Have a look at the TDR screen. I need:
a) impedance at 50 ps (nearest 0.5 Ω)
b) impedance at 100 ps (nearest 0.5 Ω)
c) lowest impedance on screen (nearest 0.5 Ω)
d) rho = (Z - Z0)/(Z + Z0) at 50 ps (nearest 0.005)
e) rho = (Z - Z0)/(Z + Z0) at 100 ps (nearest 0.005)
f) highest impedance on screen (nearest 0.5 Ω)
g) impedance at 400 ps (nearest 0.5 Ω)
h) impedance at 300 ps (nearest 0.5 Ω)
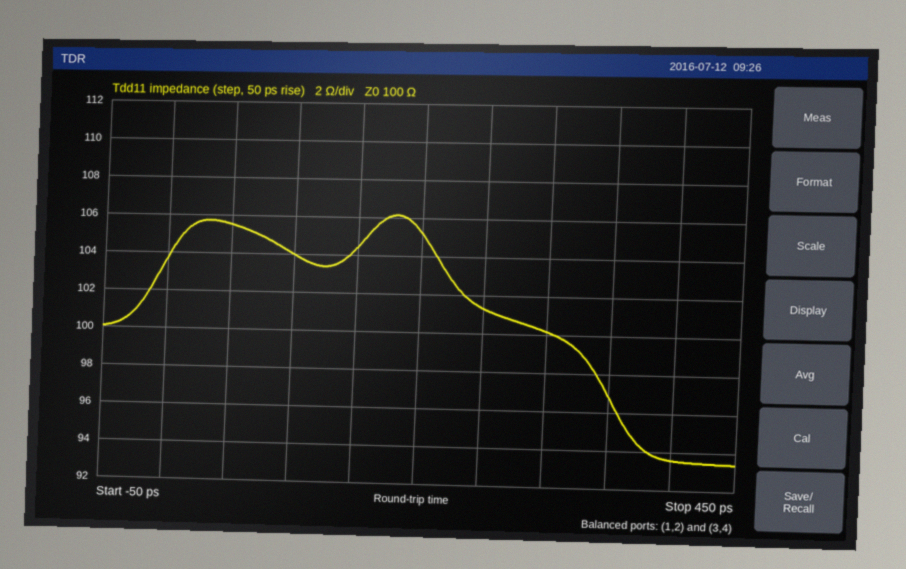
105.5 Ω
104.0 Ω
93.5 Ω
+0.025
+0.020
106.0 Ω
93.5 Ω
100.0 Ω
